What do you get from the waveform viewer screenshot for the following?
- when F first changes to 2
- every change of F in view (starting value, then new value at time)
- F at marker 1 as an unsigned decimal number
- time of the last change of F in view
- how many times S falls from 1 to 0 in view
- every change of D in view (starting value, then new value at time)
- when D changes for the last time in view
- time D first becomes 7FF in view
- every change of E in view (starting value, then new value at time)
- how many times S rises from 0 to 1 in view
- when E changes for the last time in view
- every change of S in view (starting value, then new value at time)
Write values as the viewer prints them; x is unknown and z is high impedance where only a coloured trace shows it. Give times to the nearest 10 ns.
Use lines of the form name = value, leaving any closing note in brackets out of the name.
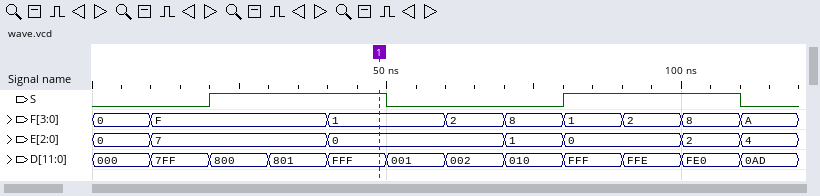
when F first changes to 2 = 60 ns
every change of F in view = 0, F at 10 ns, 1 at 40 ns, 2 at 60 ns, 8 at 70 ns, 1 at 80 ns, 2 at 90 ns, 8 at 100 ns, A at 110 ns
F at marker 1 as an unsigned decimal number = 1
time of the last change of F in view = 110 ns
how many times S falls from 1 to 0 in view = 2
every change of D in view = 000, 7FF at 10 ns, 800 at 20 ns, 801 at 30 ns, FFF at 40 ns, 001 at 50 ns, 002 at 60 ns, 010 at 70 ns, FFF at 80 ns, FFE at 90 ns, FE0 at 100 ns, 0AD at 110 ns
when D changes for the last time in view = 110 ns
time D first becomes 7FF in view = 10 ns
every change of E in view = 0, 7 at 10 ns, 0 at 40 ns, 1 at 70 ns, 0 at 80 ns, 2 at 100 ns, 4 at 110 ns
how many times S rises from 0 to 1 in view = 2
when E changes for the last time in view = 110 ns
every change of S in view = 0, 1 at 20 ns, 0 at 50 ns, 1 at 80 ns, 0 at 110 ns
